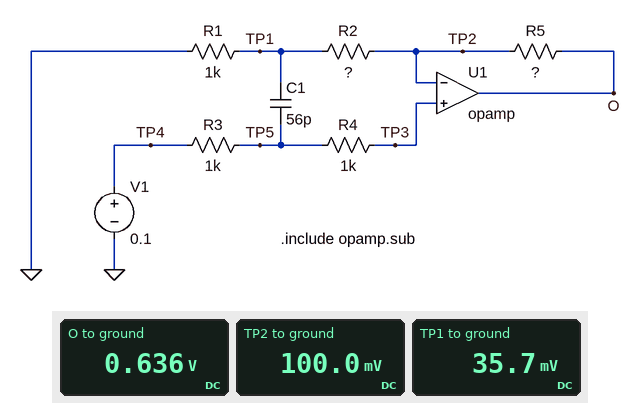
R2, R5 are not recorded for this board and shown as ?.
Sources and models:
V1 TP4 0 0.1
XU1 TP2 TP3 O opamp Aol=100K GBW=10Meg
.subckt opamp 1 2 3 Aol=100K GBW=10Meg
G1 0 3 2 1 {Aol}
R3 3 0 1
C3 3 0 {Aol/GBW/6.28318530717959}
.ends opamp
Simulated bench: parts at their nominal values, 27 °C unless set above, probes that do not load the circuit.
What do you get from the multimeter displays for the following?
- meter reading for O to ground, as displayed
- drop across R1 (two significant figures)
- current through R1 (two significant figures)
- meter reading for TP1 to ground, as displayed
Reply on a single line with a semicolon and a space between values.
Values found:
0.636 V; 36 mV; 36 µA; 35.7 mV
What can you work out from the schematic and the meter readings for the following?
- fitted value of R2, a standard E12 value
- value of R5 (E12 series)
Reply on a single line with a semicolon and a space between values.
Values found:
1.8 kΩ; 15 kΩ
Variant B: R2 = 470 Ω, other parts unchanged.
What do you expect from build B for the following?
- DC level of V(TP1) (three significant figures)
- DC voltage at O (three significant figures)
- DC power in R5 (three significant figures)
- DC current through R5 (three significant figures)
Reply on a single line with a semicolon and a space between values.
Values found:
68.0 mV; 1.12 V; 69.4 µW; 68.0 µA
